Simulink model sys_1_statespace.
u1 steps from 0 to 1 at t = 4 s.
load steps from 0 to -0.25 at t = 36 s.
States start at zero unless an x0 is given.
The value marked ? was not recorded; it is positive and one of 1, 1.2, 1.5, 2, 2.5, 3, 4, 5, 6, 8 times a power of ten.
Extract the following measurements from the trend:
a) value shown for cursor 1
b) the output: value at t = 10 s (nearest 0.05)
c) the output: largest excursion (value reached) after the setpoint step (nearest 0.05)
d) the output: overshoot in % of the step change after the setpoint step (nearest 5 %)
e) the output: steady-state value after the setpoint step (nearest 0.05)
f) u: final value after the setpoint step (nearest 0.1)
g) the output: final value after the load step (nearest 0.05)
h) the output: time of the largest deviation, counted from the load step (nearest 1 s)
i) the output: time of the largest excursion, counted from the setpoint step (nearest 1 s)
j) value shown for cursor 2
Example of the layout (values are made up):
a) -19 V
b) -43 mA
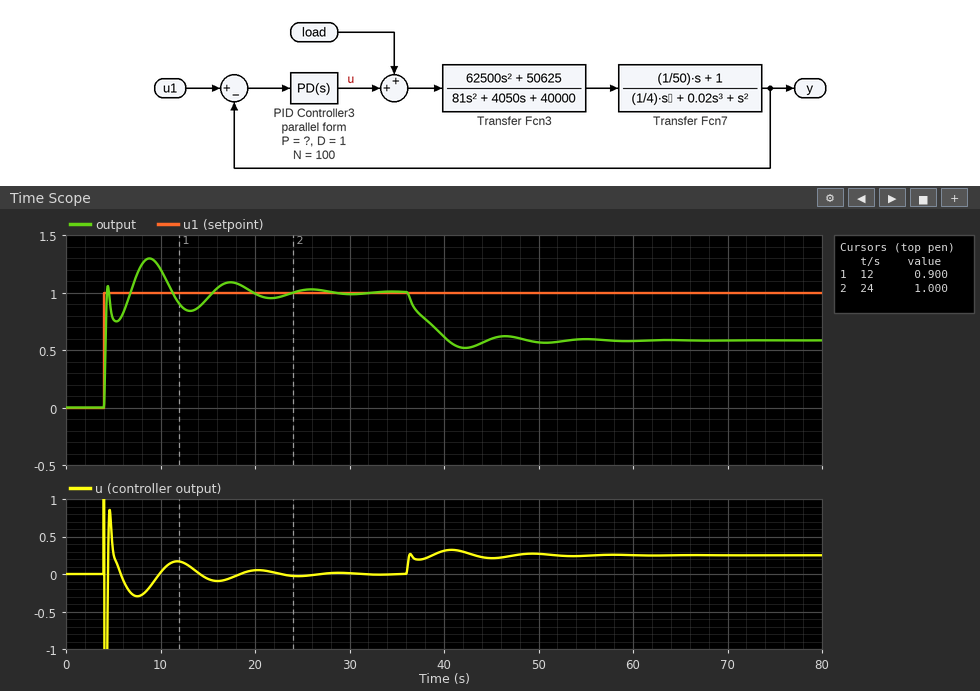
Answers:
a) 0.900
b) 1.20
c) 1.30
d) 30 %
e) 1.00
f) 0.0
g) 0.60
h) 6 s
i) 5 s
j) 1.000
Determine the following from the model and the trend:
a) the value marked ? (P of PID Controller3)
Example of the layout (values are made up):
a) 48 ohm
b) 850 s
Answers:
a) 0.6
